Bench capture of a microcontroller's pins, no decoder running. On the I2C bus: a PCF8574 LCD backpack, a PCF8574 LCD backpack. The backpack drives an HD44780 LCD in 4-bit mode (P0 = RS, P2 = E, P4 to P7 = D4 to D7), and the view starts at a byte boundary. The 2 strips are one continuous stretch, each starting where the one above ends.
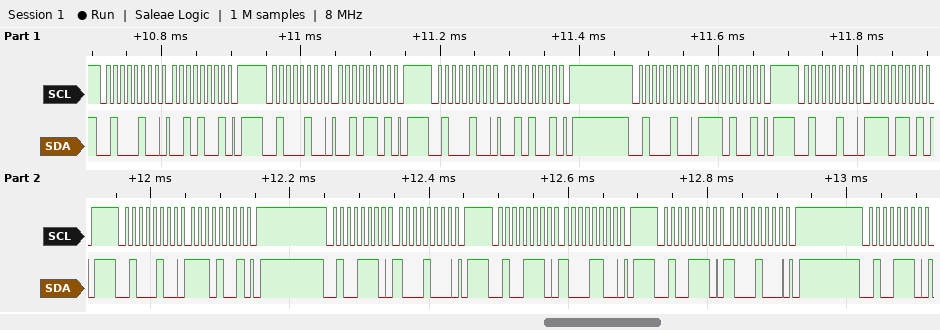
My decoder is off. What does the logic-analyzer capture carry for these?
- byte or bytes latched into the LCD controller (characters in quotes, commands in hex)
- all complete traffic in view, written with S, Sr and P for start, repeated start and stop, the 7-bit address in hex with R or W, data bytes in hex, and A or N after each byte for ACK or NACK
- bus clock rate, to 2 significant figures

'.'
S 22W A 29 A P S 22W A 2D A P S 22W A 29 A P S 22W A E9 A P S 22W A ED A P S 22W A E9 A P S 27W A 88 A P S 27W A 8C A P S 27W A 88 A P S 27W A
100 kHz
